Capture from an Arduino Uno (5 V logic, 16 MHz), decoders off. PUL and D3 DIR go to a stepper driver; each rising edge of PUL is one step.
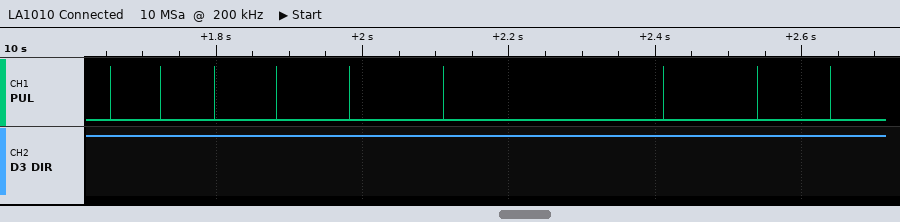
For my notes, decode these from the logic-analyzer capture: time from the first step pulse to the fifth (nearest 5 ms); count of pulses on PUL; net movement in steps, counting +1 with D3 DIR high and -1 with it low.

325 ms
9
+9
